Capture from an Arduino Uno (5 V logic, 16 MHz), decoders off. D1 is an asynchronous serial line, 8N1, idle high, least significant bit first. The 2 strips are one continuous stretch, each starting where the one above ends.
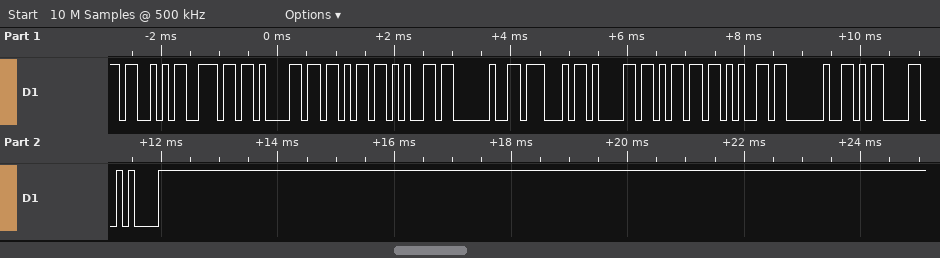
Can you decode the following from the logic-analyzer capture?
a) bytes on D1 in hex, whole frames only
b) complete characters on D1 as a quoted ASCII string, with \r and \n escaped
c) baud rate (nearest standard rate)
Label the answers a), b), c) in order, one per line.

a) 53 6E 61 6B 65 20 47 61 6D 65 20 0D 0A
b) "Snake Game \r\n"
c) 9600 baud
